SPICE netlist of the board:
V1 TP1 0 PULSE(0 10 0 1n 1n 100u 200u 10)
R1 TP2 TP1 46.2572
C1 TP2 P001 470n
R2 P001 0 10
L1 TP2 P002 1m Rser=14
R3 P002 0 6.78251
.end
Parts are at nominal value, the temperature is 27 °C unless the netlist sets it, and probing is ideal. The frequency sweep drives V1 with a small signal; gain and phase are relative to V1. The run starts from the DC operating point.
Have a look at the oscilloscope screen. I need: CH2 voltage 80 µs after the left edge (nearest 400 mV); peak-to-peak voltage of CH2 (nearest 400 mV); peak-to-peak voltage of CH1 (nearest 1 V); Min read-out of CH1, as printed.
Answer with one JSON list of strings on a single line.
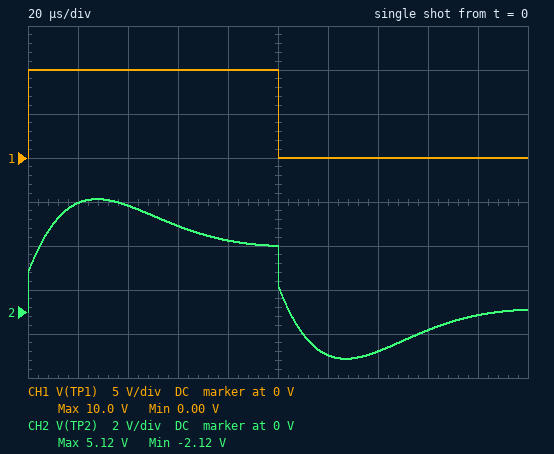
["3.2 V", "7.2 V", "10 V", "0.00 V"]
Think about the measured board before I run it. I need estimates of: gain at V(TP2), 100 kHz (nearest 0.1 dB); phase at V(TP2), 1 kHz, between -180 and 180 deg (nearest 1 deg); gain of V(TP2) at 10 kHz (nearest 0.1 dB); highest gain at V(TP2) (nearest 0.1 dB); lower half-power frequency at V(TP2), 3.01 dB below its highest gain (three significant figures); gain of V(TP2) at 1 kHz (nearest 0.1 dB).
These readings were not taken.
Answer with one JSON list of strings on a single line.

["-14.5 dB", "9 deg", "-4.6 dB", "-4.0 dB", "3.35 kHz", "-9.8 dB"]
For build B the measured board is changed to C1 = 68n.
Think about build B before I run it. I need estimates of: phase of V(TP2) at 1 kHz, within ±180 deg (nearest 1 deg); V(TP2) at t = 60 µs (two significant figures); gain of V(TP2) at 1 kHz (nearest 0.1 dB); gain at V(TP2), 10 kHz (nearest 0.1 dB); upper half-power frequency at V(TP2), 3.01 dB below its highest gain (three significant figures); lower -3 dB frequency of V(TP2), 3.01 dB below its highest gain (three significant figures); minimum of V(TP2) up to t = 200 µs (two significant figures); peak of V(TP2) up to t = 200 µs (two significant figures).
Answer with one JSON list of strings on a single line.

["11 deg", "3.2 V", "-9.8 dB", "-2.4 dB", "55.4 kHz", "7.31 kHz", "-4.6 V", "7.7 V"]
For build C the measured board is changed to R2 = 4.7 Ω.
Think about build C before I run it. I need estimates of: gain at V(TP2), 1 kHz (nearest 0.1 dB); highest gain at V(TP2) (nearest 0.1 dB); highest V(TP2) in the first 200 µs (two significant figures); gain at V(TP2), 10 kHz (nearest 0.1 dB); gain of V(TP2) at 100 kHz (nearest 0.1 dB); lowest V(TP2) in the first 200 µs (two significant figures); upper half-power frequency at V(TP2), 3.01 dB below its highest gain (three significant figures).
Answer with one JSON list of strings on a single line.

["-9.8 dB", "-3.4 dB", "5.4 V", "-3.9 dB", "-18.9 dB", "-2.4 V", "14.7 kHz"]
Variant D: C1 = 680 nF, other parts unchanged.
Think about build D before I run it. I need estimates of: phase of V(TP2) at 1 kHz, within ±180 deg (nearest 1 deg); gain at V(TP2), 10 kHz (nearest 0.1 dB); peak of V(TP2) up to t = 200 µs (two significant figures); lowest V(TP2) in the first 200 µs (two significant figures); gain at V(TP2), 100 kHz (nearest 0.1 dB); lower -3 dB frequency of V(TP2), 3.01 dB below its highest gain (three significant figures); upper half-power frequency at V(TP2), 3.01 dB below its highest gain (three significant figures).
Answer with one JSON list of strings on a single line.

["8 deg", "-6.8 dB", "4.6 V", "-1.6 V", "-14.8 dB", "2.44 kHz", "12.4 kHz"]
